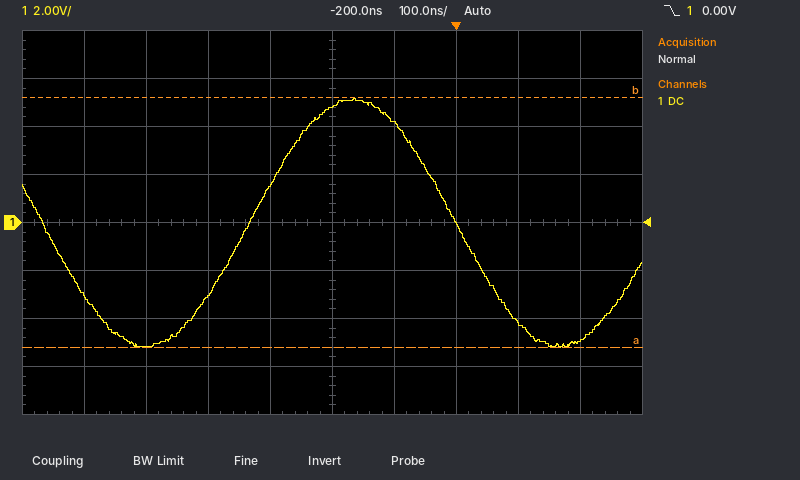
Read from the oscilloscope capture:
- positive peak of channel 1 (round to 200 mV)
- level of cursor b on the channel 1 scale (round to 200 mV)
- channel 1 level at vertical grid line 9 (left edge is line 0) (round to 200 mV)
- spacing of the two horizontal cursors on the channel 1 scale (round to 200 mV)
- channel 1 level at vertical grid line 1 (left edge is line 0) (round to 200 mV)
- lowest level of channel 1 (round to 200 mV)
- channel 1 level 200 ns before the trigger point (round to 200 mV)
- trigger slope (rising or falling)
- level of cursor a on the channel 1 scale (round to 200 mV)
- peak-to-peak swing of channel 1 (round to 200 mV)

5.2 V
5.2 V
-5.0 V
10.4 V
-3.0 V
-5.2 V
4.8 V
falling
-5.2 V
10.4 V
